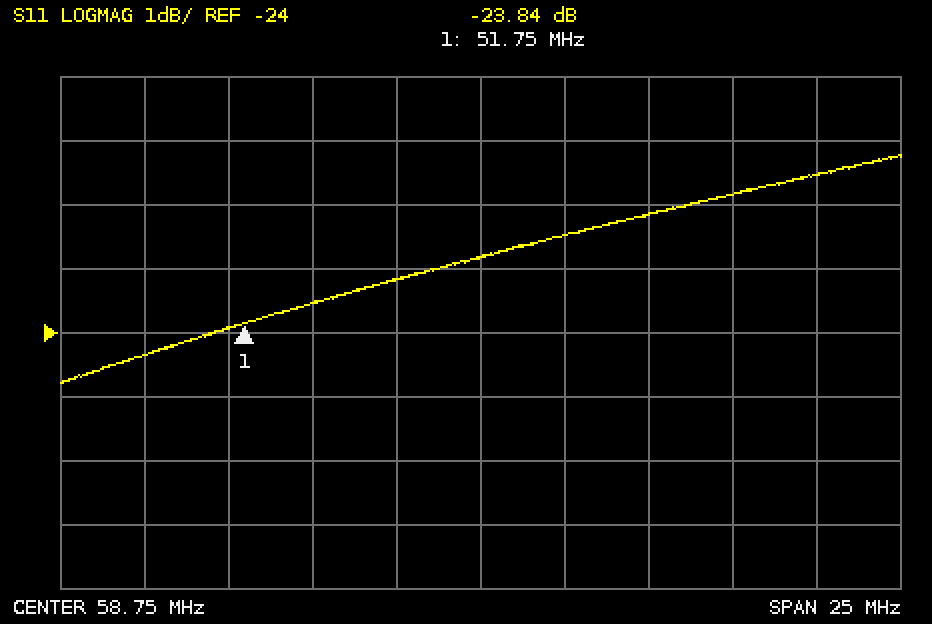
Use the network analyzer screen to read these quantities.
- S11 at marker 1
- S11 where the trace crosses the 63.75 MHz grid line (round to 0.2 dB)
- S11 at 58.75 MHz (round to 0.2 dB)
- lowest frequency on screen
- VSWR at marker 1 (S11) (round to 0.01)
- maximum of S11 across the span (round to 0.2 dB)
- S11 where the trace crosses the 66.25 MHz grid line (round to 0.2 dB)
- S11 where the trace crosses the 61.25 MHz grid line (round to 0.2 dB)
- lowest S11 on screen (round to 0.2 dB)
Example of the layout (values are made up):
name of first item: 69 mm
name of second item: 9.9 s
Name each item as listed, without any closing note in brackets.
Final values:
S11 at marker 1: -23.84 dB
S11 where the trace crosses the 63.75 MHz grid line: -22.2 dB
S11 at 58.75 MHz: -22.8 dB
lowest frequency on screen: 46.25 MHz
VSWR at marker 1 (S11): 1.14
maximum of S11 across the span: -21.2 dB
S11 where the trace crosses the 66.25 MHz grid line: -21.8 dB
S11 where the trace crosses the 61.25 MHz grid line: -22.4 dB
lowest S11 on screen: -24.8 dB
